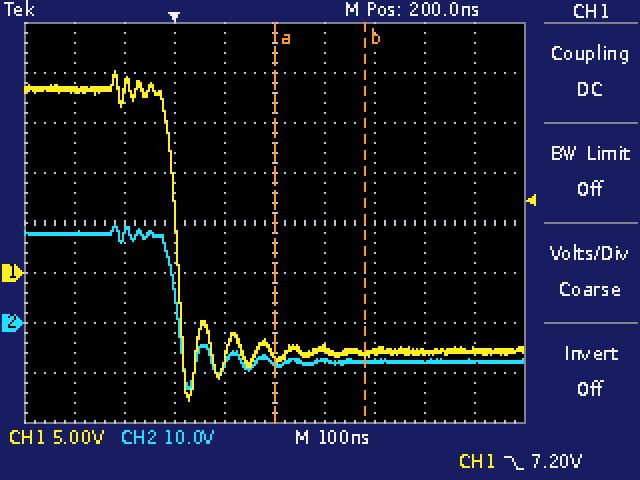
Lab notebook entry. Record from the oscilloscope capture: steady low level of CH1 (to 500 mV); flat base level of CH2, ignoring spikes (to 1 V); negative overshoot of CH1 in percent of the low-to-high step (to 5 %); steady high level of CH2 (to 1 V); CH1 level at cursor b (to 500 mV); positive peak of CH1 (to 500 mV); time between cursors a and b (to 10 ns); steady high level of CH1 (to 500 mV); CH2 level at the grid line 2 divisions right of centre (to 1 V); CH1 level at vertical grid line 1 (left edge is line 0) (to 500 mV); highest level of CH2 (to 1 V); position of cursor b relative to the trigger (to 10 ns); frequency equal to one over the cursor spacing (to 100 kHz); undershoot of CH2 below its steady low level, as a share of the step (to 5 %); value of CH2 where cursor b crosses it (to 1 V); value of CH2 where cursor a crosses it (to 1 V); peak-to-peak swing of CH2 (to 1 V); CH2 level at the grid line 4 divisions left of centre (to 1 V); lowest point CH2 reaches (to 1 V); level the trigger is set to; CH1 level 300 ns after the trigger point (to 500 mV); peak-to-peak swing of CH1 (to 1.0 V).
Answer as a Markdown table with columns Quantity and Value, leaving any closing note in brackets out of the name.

| Quantity | Value |
|---|---|
| steady low level of CH1 | -8.0 V |
| flat base level of CH2, ignoring spikes | -8 V |
| negative overshoot of CH1 in percent of the low-to-high step | 20 % |
| steady high level of CH2 | 18 V |
| CH1 level at cursor b | -8.0 V |
| positive peak of CH1 | 20.0 V |
| time between cursors a and b | 180 ns |
| steady high level of CH1 | 18.5 V |
| CH2 level at the grid line 2 divisions right of centre | -8 V |
| CH1 level at vertical grid line 1 (left edge is line 0) | 18.5 V |
| highest level of CH2 | 20 V |
| position of cursor b relative to the trigger | +380 ns |
| frequency equal to one over the cursor spacing | 5.6 MHz |
| undershoot of CH2 below its steady low level, as a share of the step | 20 % |
| value of CH2 where cursor b crosses it | -8 V |
| value of CH2 where cursor a crosses it | -8 V |
| peak-to-peak swing of CH2 | 33 V |
| CH2 level at the grid line 4 divisions left of centre | 18 V |
| lowest point CH2 reaches | -13 V |
| level the trigger is set to | 7.20 V |
| CH1 level 300 ns after the trigger point | -7.5 V |
| peak-to-peak swing of CH1 | 33.0 V |
